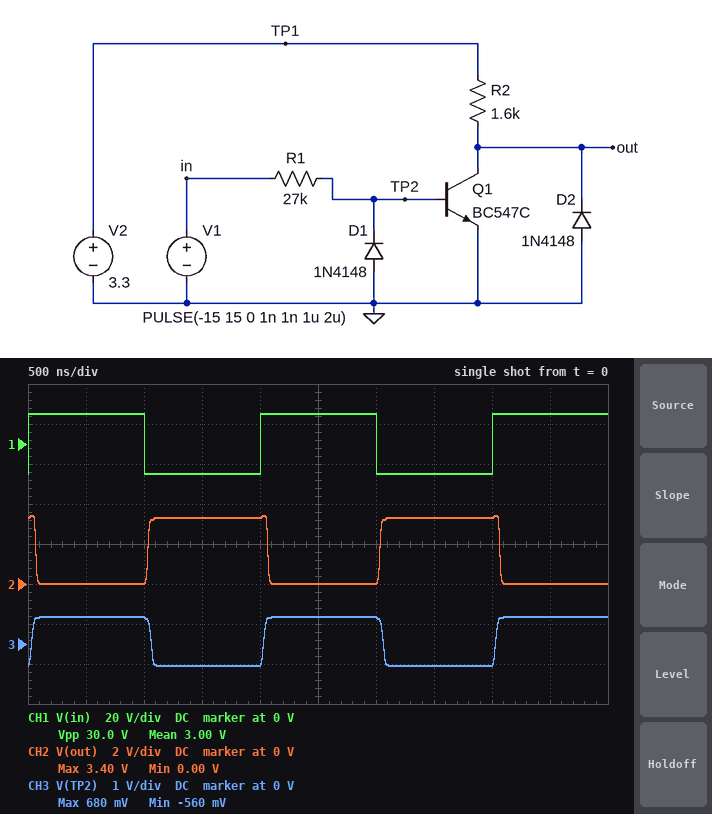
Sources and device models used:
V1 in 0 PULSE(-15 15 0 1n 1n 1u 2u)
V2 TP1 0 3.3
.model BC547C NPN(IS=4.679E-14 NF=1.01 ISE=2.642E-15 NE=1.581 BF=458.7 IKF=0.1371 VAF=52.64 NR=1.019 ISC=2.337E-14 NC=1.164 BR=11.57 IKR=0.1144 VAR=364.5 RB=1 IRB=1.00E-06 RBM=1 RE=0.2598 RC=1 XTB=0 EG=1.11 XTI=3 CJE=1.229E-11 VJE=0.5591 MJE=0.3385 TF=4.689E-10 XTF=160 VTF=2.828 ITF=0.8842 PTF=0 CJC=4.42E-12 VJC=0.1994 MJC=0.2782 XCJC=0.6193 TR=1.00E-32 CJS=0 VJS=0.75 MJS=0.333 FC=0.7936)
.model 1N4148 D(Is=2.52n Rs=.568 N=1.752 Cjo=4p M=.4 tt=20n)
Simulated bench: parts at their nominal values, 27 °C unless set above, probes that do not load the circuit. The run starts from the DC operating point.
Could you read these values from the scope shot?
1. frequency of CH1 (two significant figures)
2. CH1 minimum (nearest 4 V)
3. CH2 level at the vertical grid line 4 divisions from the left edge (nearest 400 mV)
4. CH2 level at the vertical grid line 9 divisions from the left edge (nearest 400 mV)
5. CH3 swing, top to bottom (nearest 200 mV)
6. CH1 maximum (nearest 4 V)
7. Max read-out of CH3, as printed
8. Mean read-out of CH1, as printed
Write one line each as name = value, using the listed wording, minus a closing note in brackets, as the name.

frequency of CH1 = 500 kHz
CH1 minimum = -16 V
CH2 level at the vertical grid line 4 divisions from the left edge = 3.2 V
CH2 level at the vertical grid line 9 divisions from the left edge = 0 V
CH3 swing, top to bottom = 1.2 V
CH1 maximum = 16 V
Max read-out of CH3, as printed = 680 mV
Mean read-out of CH1, as printed = 3.00 V
